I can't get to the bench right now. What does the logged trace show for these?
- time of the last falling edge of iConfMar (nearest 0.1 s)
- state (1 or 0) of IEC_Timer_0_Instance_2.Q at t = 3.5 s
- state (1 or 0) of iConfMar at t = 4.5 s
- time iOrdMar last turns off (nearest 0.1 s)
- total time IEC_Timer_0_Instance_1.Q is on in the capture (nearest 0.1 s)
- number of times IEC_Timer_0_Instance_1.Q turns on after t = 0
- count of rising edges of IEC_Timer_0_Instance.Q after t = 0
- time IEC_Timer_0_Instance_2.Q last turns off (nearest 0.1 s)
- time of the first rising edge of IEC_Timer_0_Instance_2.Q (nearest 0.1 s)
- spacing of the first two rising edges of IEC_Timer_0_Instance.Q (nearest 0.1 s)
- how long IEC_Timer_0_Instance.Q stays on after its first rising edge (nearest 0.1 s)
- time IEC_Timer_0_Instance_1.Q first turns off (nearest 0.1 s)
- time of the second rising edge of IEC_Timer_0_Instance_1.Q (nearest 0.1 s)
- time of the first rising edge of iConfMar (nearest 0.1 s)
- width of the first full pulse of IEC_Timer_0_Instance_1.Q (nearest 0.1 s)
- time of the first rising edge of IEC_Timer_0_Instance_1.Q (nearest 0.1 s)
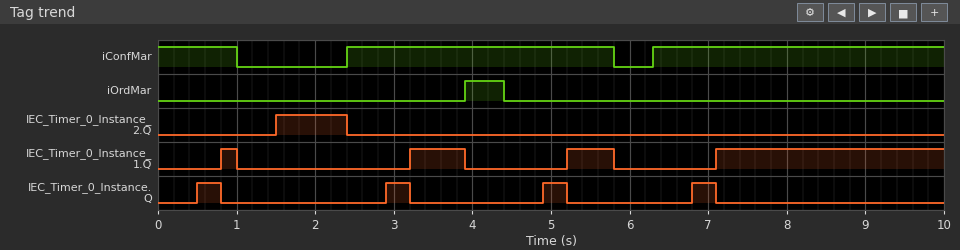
5.8 s
0
1
4.4 s
4.4 s
4
4
2.4 s
1.5 s
2.4 s
0.3 s
1.0 s
3.2 s
2.4 s
0.2 s
0.8 s
